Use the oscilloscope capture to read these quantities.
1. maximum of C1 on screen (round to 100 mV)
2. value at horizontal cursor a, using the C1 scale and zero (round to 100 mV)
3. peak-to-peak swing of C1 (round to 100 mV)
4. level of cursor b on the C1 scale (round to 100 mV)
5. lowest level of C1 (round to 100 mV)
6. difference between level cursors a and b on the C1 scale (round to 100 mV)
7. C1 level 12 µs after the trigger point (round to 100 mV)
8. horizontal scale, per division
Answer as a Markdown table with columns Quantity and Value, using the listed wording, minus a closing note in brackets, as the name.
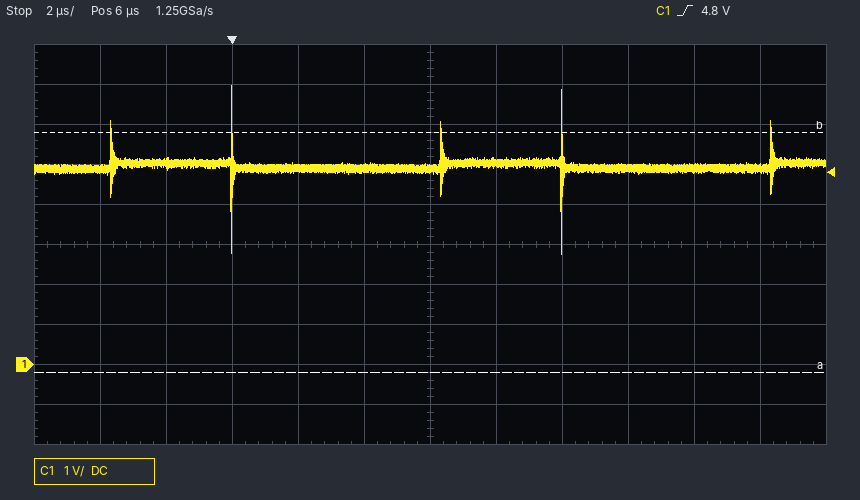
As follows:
| Quantity | Value |
|---|---|
| maximum of C1 on screen | 7.0 V |
| value at horizontal cursor a, using the C1 scale and zero | -200 mV |
| peak-to-peak swing of C1 | 4.2 V |
| level of cursor b on the C1 scale | 5.8 V |
| lowest level of C1 | 2.8 V |
| difference between level cursors a and b on the C1 scale | 6.0 V |
| C1 level 12 µs after the trigger point | 4.9 V |
| horizontal scale, per division | 2 µs |
